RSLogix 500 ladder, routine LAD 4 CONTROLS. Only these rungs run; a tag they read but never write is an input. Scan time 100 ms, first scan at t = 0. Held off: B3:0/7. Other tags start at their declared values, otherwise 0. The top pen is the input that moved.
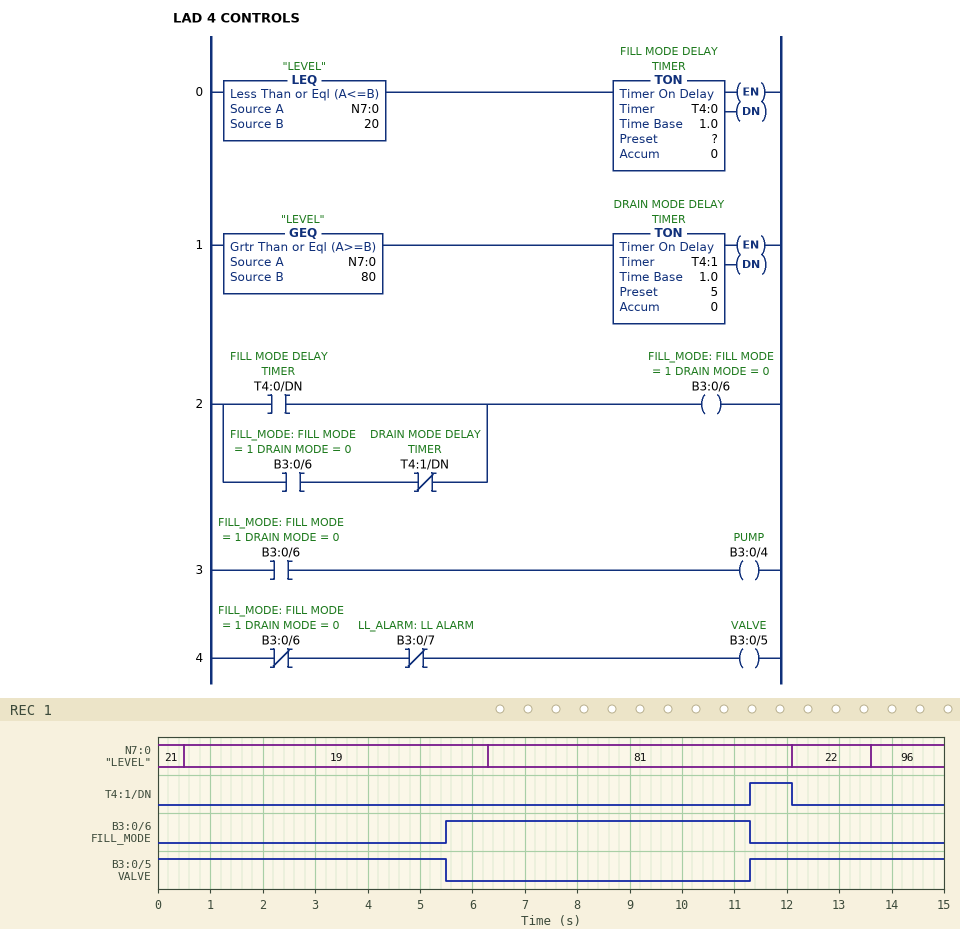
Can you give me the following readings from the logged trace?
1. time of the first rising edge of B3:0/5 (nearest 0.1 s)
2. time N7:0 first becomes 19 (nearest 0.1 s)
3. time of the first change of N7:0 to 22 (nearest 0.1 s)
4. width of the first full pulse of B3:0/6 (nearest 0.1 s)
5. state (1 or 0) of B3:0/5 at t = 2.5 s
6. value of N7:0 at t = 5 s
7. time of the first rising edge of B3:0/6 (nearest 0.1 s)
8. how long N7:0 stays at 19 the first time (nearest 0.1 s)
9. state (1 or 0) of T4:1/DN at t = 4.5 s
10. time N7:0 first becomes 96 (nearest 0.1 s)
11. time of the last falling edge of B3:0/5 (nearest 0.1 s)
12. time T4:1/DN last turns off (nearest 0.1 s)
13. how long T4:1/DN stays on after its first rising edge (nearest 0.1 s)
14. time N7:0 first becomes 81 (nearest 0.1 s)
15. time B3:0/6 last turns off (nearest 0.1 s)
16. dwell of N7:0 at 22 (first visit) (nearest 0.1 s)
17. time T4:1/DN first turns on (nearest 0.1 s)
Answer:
11.3 s
0.5 s
12.1 s
5.8 s
1
19
5.5 s
5.8 s
0
13.6 s
5.5 s
12.1 s
0.8 s
6.3 s
11.3 s
1.5 s
11.3 s
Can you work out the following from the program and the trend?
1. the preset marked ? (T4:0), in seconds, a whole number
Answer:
5 s
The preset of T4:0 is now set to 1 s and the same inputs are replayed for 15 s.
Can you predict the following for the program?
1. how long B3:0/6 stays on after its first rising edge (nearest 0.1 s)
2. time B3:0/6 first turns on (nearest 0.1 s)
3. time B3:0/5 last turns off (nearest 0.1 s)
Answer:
9.8 s
1.5 s
1.5 s
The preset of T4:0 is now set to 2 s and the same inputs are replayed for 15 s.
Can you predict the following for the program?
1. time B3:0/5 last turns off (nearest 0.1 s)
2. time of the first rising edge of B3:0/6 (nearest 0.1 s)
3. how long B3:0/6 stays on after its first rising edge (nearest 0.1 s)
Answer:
2.5 s
2.5 s
8.8 s
